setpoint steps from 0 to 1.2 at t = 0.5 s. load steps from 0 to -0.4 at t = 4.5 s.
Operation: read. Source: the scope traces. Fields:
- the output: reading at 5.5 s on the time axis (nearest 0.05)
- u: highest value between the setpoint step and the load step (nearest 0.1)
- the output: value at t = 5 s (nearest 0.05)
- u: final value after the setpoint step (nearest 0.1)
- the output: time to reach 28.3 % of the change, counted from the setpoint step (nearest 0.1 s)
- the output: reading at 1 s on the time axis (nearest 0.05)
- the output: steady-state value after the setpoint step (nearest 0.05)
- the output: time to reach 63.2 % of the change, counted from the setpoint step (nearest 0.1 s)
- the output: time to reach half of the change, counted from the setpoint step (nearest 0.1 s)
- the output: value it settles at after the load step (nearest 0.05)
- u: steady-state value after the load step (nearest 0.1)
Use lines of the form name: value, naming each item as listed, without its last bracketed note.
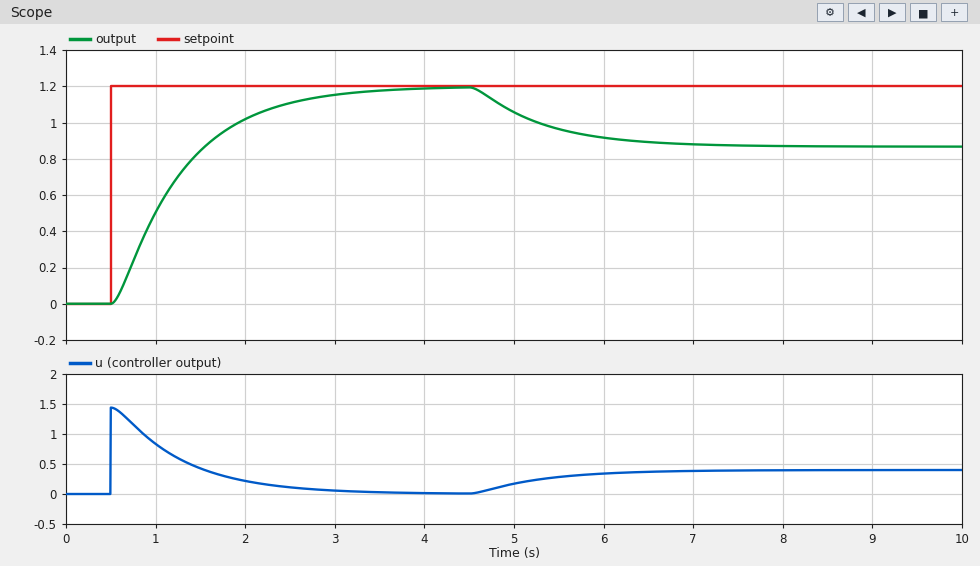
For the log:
the output: reading at 5.5 s on the time axis: 0.95
u: highest value between the setpoint step and the load step: 1.4
the output: value at t = 5 s: 1.05
u: final value after the setpoint step: 0.0
the output: time to reach 28.3 % of the change, counted from the setpoint step: 0.3 s
the output: reading at 1 s on the time axis: 0.50
the output: steady-state value after the setpoint step: 1.20
the output: time to reach 63.2 % of the change, counted from the setpoint step: 0.8 s
the output: time to reach half of the change, counted from the setpoint step: 0.6 s
the output: value it settles at after the load step: 0.85
u: steady-state value after the load step: 0.4
